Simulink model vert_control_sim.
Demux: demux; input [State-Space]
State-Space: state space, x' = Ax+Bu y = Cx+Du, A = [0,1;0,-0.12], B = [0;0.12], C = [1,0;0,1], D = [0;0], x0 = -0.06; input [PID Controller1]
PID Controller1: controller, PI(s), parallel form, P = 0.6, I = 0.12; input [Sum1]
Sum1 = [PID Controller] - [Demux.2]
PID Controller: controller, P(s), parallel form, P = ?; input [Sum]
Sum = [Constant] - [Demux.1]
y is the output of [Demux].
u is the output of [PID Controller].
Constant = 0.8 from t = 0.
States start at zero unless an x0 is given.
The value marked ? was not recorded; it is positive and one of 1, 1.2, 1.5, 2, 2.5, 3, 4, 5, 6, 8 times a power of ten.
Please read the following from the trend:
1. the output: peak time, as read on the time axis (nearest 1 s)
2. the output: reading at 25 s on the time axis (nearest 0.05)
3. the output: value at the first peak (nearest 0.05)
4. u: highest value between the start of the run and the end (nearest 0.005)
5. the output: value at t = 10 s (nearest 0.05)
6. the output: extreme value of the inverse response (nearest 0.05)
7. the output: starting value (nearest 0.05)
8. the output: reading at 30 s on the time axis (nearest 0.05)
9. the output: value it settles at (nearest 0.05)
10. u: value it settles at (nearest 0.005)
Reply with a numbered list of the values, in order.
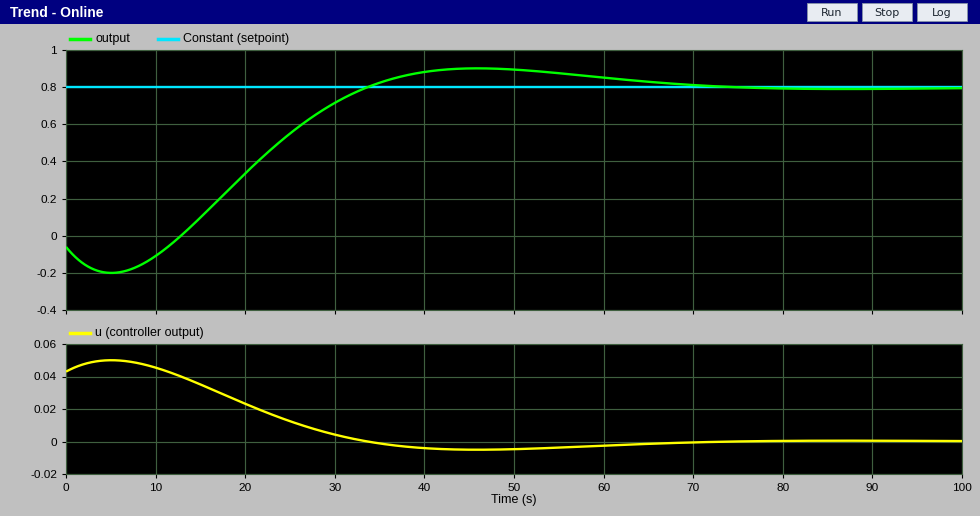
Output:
1. 46 s
2. 0.55
3. 0.90
4. 0.050
5. -0.10
6. -0.20
7. -0.05
8. 0.70
9. 0.80
10. 0.000
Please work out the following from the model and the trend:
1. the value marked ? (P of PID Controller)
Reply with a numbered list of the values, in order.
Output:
1. 0.05
